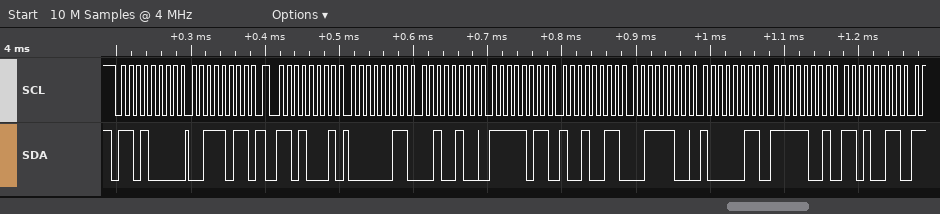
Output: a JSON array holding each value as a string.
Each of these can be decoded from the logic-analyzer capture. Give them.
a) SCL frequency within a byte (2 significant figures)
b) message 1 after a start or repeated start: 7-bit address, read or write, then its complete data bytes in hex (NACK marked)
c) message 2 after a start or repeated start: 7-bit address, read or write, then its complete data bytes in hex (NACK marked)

["100 kHz", "0x68 write: 3B", "0x68 read: 03 24 FB 93 3C 83 F9 D3"]
